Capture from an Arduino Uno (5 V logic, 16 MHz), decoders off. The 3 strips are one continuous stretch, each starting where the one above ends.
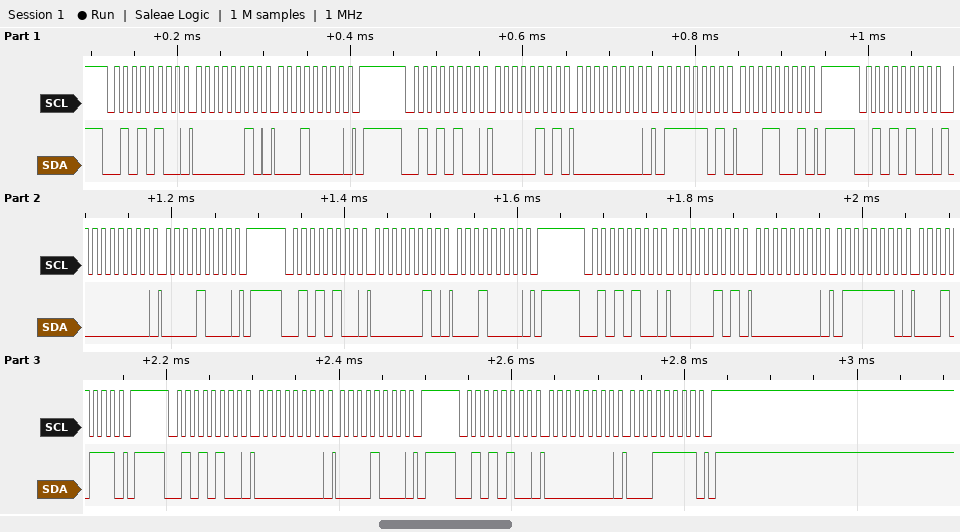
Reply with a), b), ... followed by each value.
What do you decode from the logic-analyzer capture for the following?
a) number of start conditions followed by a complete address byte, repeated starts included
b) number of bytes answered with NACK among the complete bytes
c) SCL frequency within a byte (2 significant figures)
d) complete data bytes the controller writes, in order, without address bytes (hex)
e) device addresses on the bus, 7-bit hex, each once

a) 7
b) 0
c) 100 kHz
d) 02 10 05 00 7D 19 00 08 02 10 05 00 7E 17 00 08 00 1F
e) 0x2A
